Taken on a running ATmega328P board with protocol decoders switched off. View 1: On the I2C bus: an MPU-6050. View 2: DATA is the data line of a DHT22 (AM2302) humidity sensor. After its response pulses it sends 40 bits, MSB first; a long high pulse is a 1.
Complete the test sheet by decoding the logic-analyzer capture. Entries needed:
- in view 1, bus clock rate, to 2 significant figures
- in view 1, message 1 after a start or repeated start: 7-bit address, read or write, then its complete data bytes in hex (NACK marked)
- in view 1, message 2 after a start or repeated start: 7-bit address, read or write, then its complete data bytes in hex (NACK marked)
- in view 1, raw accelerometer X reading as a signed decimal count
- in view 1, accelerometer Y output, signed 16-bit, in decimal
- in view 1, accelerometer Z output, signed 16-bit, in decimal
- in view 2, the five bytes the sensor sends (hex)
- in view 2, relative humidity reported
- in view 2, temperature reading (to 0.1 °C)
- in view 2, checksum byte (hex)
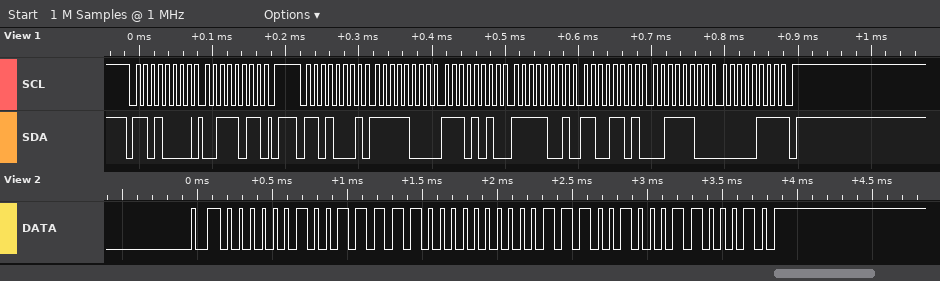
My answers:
100 kHz
0x68 write: 3B
0x68 read: F8 EA F9 CD 3C 07 NACK
-1814
-1587
15367
02 7C 00 E4 62
63.6 %
22.8 °C
0x62
